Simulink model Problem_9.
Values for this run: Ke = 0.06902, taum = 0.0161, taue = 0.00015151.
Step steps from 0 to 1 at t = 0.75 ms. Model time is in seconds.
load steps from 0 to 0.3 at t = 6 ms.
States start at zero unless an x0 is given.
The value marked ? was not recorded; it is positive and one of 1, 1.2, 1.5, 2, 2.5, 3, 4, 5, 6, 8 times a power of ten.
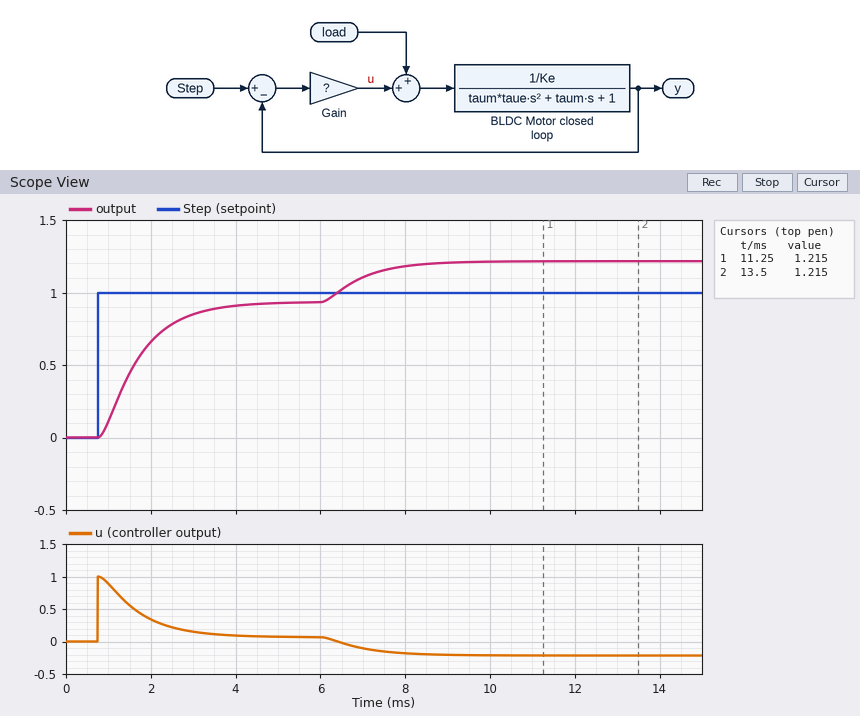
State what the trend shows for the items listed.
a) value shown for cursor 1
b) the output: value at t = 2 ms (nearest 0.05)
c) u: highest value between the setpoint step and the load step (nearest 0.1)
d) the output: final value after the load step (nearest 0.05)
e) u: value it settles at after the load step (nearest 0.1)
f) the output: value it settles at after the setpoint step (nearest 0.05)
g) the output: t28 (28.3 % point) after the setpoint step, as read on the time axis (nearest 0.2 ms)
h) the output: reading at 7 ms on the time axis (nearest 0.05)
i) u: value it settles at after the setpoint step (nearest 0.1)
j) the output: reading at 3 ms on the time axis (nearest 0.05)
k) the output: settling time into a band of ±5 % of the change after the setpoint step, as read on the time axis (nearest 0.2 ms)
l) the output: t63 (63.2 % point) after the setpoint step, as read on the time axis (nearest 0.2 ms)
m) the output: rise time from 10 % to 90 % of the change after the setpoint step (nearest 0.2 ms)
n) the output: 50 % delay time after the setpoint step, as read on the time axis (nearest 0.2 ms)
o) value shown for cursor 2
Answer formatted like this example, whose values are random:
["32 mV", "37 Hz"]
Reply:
["1.215", "0.65", "1.0", "1.20", "-0.2", "0.95", "1.2 ms", "1.10", "0.1", "0.85", "3.6 ms", "1.8 ms", "2.0 ms", "1.6 ms", "1.215"]
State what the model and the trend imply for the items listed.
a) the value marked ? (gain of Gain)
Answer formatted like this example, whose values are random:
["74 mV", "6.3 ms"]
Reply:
["1"]
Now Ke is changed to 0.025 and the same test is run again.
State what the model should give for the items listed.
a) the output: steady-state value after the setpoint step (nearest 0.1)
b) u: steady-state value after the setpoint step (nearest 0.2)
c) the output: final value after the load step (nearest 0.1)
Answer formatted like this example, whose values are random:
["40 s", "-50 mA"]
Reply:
["1.0", "0.0", "1.3"]
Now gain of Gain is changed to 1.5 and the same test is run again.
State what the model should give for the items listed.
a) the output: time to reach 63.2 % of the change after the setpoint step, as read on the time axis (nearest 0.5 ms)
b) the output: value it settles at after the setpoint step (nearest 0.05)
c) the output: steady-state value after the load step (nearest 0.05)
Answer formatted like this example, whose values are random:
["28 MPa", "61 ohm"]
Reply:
["1.5 ms", "0.95", "1.15"]
